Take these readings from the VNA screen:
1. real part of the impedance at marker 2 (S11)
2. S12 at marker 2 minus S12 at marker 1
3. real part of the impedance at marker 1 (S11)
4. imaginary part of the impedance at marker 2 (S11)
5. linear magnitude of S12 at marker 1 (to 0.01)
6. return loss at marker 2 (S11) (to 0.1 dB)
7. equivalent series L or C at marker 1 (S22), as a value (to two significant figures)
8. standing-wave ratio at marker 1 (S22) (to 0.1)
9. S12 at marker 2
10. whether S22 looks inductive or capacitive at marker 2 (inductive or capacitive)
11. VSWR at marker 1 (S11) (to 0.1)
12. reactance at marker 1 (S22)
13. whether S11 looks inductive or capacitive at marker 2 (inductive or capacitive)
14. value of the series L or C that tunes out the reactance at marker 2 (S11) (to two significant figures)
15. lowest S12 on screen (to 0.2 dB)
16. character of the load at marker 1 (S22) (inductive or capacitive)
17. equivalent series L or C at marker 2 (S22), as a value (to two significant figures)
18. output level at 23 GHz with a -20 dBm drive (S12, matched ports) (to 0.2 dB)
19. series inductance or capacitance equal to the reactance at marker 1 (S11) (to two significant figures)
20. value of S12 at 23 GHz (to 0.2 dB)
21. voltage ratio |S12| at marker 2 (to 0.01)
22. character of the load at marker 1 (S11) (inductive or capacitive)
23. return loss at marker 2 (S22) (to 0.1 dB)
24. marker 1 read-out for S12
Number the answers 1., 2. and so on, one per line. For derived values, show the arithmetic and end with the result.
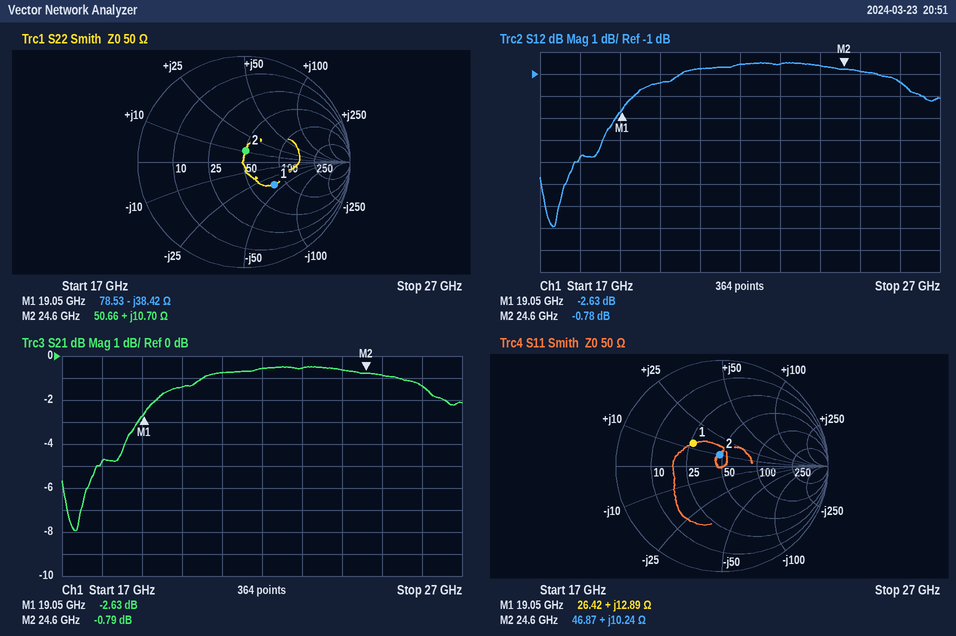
1. 46.87 Ω
2. -0.78 − (-2.63) = 1.85 dB
3. 26.42 Ω
4. +10.24 Ω
5. 10^(-2.63/20) ≈ 0.74
6. 19.2 dB
7. C = 1/(2π × 19.05 GHz × 38.42 Ω) ≈ 217 fF, so 220 fF to two significant figures
8. 2.1
9. -0.78 dB
10. inductive
11. 2.1
12. -38.42 Ω
13. inductive
14. C = 1/(2π × 24.6 GHz × 10.24 Ω) ≈ 632 fF, so 630 fF to two significant figures
15. -8.0 dB
16. capacitive
17. L = 10.7 Ω/(2π × 24.6 GHz) ≈ 69 pH
18. -20 dBm + (-0.6 dB) = -20.6 dBm
19. L = 12.89 Ω/(2π × 19.05 GHz) ≈ 108 pH, so 110 pH to two significant figures
20. -0.6 dB
21. 10^(-0.78/20) ≈ 0.91
22. inductive
23. 19.5 dB
24. -2.63 dB
